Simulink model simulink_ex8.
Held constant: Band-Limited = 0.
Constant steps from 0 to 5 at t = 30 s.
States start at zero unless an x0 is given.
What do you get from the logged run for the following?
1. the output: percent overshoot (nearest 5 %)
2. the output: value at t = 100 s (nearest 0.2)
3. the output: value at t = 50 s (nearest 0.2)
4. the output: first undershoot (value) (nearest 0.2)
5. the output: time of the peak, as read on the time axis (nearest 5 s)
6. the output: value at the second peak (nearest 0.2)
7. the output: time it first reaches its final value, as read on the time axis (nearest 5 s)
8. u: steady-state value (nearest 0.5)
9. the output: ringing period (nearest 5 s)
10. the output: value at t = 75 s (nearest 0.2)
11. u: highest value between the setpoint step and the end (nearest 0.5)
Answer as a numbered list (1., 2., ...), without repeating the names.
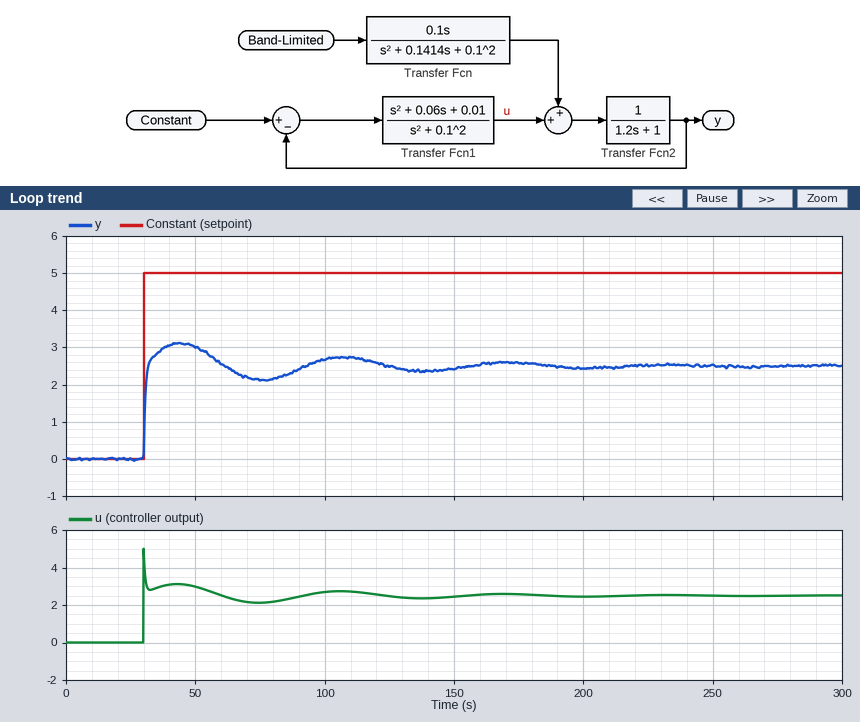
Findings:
1. 25 %
2. 2.6
3. 3.0
4. 2.2
5. 45 s
6. 2.8
7. 30 s
8. 2.5
9. 65 s
10. 2.2
11. 5.0
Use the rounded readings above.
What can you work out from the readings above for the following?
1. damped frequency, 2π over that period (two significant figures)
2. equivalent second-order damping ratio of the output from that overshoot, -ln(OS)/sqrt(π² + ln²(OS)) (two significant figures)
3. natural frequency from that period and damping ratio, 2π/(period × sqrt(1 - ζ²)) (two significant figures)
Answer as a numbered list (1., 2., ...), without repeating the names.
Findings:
1. 0.097 rad/s
2. 0.40
3. 0.11 rad/s
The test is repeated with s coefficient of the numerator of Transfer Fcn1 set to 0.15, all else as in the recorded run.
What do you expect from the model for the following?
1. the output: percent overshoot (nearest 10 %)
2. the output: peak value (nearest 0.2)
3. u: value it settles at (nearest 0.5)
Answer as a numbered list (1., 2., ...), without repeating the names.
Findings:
1. 50 %
2. 3.6
3. 2.5
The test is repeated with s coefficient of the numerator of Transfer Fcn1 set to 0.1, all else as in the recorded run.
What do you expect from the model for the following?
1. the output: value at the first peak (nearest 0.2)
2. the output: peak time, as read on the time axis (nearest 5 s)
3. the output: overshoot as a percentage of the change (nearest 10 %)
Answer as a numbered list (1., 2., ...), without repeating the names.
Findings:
1. 3.4
2. 45 s
3. 40 %
